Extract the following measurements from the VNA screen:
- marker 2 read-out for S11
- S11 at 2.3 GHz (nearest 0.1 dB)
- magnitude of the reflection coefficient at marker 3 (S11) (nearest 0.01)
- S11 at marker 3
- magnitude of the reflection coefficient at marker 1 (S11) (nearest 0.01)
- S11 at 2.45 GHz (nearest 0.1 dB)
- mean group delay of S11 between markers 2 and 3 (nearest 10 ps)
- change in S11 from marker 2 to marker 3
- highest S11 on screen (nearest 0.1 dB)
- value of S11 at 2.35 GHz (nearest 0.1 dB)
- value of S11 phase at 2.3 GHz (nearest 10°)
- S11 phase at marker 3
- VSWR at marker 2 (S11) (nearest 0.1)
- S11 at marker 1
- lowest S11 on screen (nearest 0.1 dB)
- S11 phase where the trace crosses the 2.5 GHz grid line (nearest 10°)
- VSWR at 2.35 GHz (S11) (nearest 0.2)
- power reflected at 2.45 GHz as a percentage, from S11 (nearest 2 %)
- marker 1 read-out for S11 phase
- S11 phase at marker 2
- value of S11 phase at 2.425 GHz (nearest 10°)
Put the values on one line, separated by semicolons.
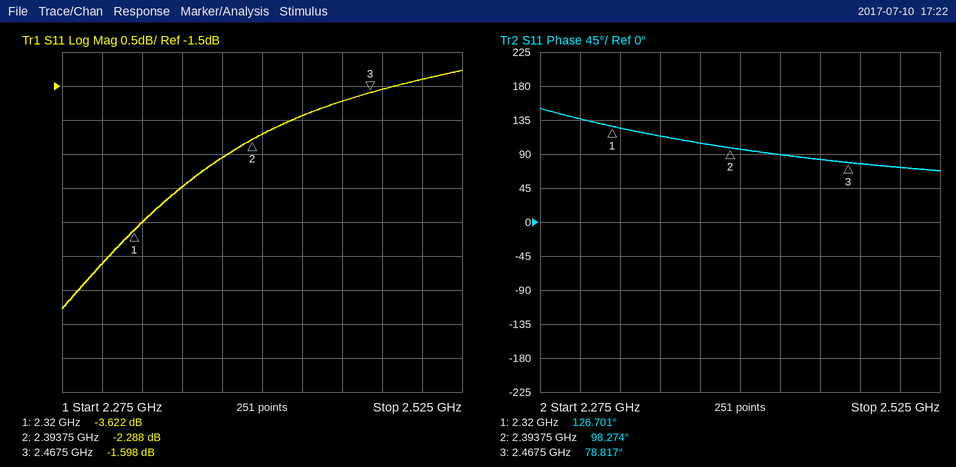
-2.288 dB; -4.1 dB; 0.83; -1.598 dB; 0.66; -1.7 dB; 730 ps; 0.690 dB; -1.3 dB; -3.0 dB; 140°; 78.817°; 7.6; -3.622 dB; -4.8 dB; 70°; 5.8; 68 %; 126.701°; 98.274°; 90°
